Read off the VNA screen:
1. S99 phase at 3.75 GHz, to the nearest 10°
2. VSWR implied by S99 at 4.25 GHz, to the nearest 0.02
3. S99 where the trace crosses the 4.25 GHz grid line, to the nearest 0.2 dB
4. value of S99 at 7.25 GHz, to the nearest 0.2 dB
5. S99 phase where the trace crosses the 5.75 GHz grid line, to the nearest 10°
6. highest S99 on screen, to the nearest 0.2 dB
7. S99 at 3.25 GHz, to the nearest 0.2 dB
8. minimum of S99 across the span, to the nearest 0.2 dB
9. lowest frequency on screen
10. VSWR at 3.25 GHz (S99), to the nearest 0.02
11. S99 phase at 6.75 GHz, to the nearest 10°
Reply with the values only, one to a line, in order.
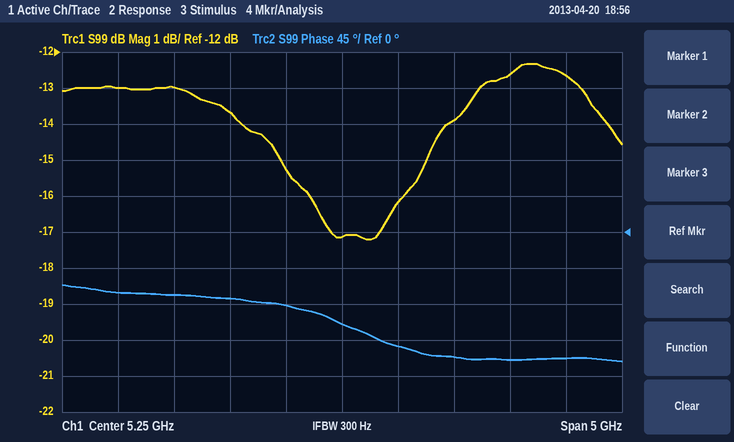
-80°
1.52
-13.6 dB
-12.6 dB
-140°
-12.4 dB
-13.0 dB
-17.2 dB
2.75 GHz
1.58
-160°
